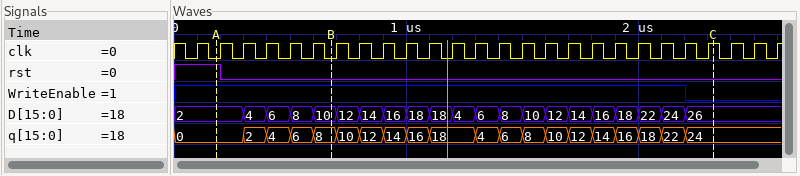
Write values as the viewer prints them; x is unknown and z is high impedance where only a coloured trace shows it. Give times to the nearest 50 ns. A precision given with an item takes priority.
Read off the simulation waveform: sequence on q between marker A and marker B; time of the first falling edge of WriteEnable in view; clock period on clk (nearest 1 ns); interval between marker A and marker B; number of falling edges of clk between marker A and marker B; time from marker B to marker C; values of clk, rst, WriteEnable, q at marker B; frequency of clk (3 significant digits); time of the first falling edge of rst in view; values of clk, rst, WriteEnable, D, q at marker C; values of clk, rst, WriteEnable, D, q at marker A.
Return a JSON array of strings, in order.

["0, 2, 4, 6, 8", "2200 ns", "100 ns", "500 ns", "5", "1650 ns", "clk=0, rst=0, WriteEnable=1, q=8", "10.0 MHz", "200 ns", "clk=1, rst=0, WriteEnable=0, D=26, q=24", "clk=0, rst=1, WriteEnable=1, D=2, q=0"]
